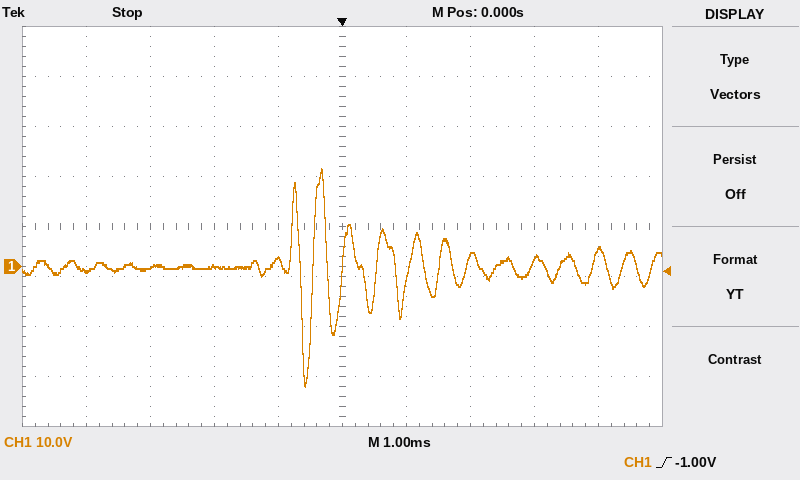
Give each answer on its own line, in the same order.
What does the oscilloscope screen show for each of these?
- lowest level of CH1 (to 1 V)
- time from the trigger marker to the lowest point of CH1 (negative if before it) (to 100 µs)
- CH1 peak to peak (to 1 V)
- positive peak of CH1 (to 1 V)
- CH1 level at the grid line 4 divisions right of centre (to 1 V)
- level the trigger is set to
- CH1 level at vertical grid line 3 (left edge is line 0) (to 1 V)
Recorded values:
-24 V
-600 µs
44 V
20 V
3 V
-1.00 V
0 V
